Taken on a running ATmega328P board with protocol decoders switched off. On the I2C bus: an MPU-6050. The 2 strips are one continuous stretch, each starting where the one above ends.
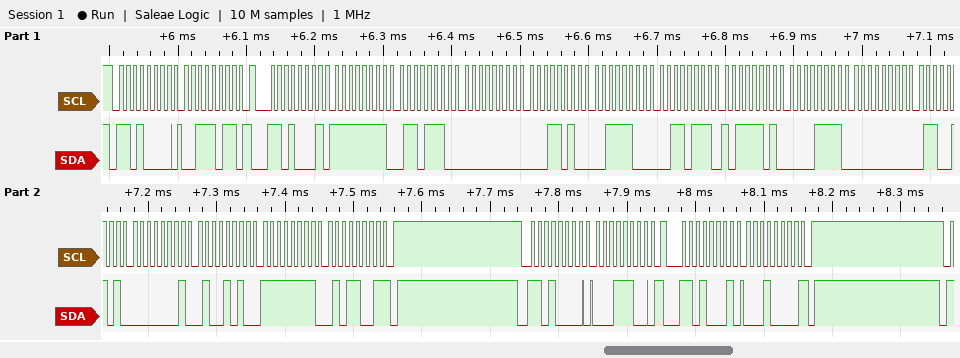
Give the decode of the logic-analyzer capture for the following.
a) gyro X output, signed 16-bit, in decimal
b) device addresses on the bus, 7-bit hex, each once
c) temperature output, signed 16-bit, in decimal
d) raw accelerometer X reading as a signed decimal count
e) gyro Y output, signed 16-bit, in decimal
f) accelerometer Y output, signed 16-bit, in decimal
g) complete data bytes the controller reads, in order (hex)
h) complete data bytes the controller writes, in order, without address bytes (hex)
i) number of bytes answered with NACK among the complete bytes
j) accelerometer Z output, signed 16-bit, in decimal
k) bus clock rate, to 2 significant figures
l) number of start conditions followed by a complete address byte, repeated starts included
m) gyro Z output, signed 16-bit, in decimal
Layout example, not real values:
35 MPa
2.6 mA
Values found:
101
0x68
-17137
-146
330
26
FF 6E 00 1A 3C 37 BD 0F 00 65 01 4A FF 59 10
3B 1C
2
15415
100 kHz
4
-167
